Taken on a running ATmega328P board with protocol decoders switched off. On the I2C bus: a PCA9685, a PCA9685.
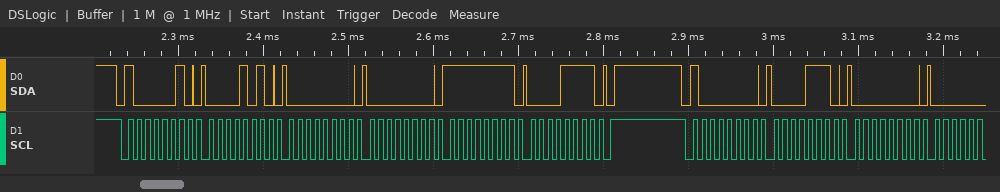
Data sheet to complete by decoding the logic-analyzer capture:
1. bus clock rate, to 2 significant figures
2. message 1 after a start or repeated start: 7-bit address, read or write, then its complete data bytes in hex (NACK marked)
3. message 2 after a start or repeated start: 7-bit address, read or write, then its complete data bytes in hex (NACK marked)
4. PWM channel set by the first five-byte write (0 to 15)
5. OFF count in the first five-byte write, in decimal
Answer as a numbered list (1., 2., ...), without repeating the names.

1. 100 kHz
2. 0x41 write: 0A 00 00 FF 0F
3. 0x40 write: 0E 00
4. 1
5. 4095
